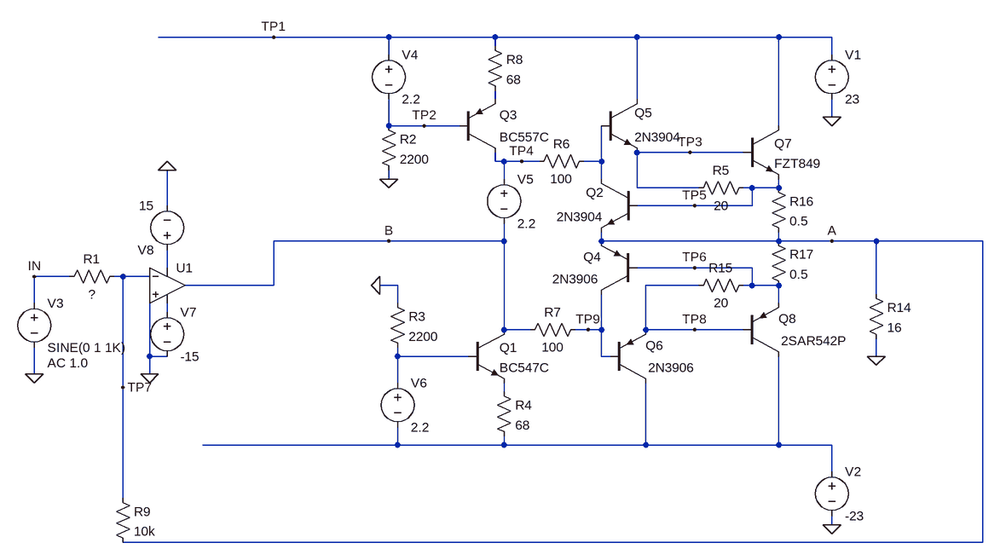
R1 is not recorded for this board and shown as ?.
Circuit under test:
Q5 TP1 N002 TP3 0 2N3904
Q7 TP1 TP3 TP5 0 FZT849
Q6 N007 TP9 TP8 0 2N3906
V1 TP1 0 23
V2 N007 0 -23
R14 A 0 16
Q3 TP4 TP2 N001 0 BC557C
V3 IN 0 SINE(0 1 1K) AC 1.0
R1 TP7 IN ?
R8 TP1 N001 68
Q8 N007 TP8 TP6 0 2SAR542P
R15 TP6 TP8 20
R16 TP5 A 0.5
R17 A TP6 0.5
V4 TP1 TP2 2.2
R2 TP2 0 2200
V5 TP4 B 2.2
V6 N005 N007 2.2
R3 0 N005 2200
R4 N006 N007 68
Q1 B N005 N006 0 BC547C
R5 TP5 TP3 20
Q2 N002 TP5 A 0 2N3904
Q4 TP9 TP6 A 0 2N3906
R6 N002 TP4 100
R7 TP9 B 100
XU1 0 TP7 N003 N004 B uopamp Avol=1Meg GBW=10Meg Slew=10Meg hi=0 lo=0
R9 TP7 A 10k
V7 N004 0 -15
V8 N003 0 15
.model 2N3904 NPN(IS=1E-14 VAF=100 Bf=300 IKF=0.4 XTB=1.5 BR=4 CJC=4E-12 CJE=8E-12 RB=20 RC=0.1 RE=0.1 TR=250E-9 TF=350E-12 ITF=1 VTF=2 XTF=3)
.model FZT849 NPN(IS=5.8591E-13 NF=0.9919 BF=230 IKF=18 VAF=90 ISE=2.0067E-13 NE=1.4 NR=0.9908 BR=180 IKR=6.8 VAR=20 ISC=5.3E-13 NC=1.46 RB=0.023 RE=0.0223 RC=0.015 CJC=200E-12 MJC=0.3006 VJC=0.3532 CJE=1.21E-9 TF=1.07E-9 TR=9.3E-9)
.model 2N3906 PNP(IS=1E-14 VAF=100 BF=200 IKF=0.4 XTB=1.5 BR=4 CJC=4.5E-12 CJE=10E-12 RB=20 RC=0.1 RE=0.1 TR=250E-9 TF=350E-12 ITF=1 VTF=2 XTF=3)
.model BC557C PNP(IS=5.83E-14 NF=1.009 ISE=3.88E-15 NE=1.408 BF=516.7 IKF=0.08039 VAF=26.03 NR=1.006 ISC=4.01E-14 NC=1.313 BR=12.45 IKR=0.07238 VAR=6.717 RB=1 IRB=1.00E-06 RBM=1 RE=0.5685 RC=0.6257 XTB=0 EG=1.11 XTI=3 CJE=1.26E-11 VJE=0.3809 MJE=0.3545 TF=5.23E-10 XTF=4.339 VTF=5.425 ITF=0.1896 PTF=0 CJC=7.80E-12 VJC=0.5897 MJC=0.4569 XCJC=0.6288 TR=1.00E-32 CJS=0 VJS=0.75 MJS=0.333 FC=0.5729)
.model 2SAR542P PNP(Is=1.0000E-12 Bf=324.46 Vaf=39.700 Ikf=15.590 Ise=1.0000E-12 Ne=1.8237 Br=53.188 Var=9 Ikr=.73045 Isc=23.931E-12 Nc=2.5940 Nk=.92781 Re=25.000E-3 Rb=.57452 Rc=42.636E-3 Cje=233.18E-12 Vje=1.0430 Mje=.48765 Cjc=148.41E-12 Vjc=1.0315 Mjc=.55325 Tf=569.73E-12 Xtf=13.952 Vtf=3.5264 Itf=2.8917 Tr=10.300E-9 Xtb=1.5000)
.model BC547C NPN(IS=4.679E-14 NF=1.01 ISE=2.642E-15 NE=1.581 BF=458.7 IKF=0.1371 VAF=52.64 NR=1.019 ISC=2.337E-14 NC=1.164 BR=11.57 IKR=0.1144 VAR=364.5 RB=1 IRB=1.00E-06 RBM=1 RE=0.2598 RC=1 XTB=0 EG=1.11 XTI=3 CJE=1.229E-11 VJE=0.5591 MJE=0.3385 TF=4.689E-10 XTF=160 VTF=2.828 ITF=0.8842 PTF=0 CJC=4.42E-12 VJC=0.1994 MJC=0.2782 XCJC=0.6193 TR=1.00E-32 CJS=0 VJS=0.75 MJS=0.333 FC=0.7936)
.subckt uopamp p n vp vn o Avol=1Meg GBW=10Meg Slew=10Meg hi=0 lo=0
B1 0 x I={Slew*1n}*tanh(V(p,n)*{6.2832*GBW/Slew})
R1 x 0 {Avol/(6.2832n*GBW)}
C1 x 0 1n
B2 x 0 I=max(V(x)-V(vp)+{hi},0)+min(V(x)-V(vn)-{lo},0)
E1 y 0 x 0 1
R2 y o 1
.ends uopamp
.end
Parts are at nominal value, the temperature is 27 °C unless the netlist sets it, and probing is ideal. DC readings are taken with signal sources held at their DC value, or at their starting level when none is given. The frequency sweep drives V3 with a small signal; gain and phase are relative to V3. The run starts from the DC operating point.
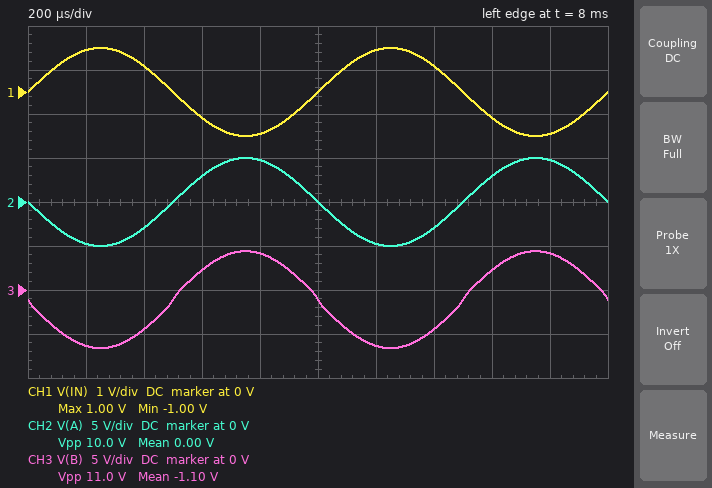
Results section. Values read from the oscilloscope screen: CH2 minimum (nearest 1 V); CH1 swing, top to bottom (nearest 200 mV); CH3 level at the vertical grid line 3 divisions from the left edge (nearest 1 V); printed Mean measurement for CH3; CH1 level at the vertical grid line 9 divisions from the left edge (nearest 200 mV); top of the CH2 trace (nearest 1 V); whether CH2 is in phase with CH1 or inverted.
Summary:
-5 V
2.0 V
2 V
-1.10 V
-1.0 V
5 V
inverted
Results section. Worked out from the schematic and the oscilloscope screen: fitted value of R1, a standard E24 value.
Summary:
2 kΩ
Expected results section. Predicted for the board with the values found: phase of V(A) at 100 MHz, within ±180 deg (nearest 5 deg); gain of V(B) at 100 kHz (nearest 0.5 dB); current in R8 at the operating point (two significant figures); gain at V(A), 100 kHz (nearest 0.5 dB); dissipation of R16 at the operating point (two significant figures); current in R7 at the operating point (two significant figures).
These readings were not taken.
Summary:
25 deg
18.5 dB
22 mA
14.0 dB
160 µW
75 µA
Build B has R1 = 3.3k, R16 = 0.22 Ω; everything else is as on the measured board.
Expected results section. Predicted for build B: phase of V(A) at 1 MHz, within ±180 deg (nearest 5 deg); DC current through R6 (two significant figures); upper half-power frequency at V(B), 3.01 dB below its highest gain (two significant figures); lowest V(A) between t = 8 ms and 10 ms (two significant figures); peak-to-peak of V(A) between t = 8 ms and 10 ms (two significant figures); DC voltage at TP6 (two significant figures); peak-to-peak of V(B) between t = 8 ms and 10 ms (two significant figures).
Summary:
145 deg
51 µA
1.4 MHz
-3.0 V
6.1 V
-9.0 mV
6.9 V
